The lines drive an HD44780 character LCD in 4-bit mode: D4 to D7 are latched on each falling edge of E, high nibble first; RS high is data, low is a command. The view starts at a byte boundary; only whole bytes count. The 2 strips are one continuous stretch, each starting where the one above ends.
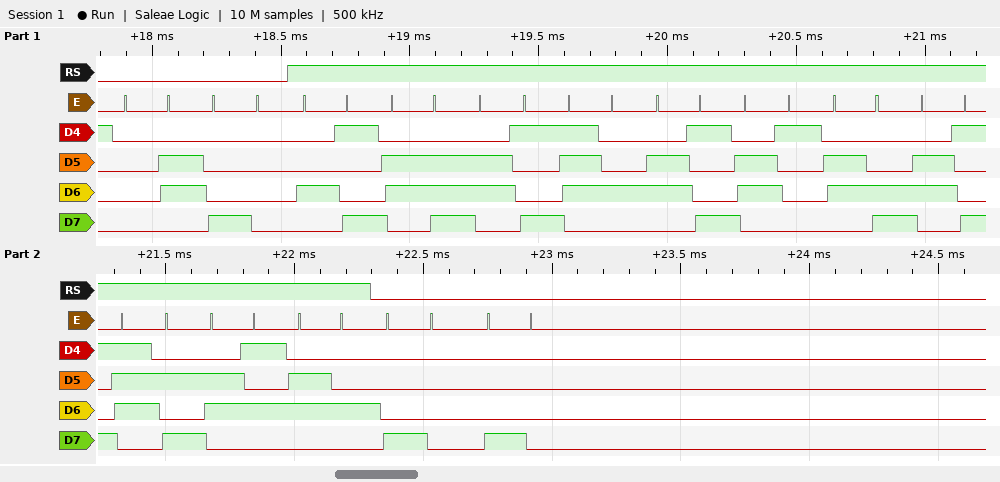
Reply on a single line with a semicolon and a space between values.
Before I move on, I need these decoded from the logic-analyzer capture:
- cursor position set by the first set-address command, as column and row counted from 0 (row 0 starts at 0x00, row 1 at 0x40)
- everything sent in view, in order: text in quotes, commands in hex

column 0, row 0; 0x06 0x80 "Initialized" 0x80 0x80
